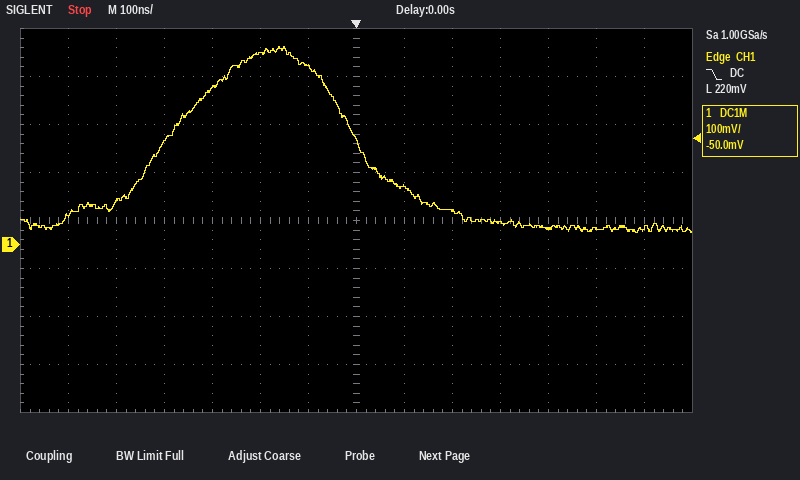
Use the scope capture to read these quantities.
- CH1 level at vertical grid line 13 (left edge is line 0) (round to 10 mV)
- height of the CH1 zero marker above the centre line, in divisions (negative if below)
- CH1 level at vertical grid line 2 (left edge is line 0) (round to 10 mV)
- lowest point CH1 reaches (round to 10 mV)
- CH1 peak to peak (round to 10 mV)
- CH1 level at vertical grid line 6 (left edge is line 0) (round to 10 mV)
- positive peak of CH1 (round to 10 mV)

30 mV
-0.5 div
90 mV
20 mV
390 mV
370 mV
410 mV
